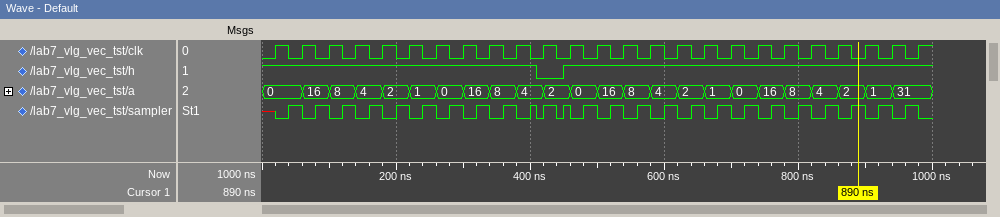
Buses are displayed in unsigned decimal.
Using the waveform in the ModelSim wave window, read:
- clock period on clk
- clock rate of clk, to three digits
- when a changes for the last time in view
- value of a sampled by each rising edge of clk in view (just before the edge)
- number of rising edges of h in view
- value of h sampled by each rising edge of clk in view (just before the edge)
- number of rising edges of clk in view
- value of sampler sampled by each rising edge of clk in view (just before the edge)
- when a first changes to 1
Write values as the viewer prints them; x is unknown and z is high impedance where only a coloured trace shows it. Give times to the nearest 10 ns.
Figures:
40 ns
25.0 MHz
940 ns
0, 0, 16, 8, 4, 2, 1, 0, 16, 8, 4, 2, 0, 16, 8, 4, 2, 1, 0, 16, 8, 4, 2, 1, 31
1
1 1 1 1 1 1 1 1 1 1 0 1 1 1 1 1 1 1 1 1 1 1 1 1 1
25
x 1 1 1 1 1 1 1 1 1 0 1 1 1 1 1 1 1 1 1 1 1 1 1 1
220 ns
